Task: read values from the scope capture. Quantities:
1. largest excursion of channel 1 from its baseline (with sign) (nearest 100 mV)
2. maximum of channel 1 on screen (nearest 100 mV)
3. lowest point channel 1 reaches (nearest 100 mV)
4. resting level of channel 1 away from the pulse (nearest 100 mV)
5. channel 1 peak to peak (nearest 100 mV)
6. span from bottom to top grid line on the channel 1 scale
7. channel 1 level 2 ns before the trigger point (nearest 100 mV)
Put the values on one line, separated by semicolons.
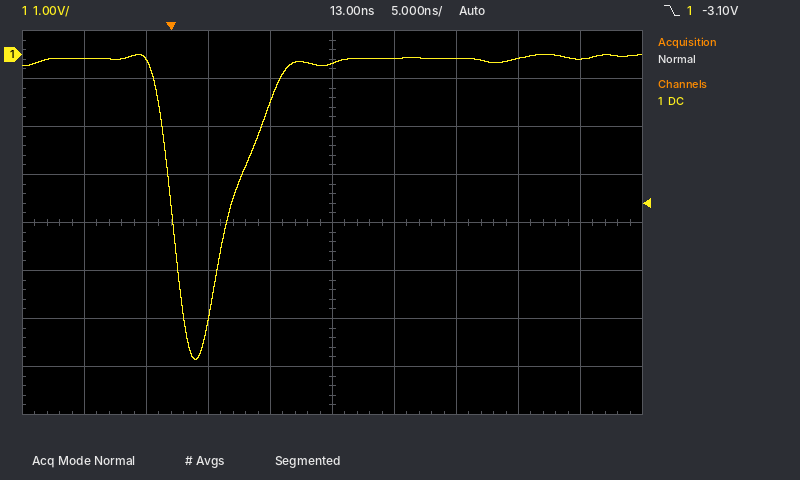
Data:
-6.3 V; 0.0 V; -6.4 V; -100 mV; 6.4 V; 8 V; -100 mV
